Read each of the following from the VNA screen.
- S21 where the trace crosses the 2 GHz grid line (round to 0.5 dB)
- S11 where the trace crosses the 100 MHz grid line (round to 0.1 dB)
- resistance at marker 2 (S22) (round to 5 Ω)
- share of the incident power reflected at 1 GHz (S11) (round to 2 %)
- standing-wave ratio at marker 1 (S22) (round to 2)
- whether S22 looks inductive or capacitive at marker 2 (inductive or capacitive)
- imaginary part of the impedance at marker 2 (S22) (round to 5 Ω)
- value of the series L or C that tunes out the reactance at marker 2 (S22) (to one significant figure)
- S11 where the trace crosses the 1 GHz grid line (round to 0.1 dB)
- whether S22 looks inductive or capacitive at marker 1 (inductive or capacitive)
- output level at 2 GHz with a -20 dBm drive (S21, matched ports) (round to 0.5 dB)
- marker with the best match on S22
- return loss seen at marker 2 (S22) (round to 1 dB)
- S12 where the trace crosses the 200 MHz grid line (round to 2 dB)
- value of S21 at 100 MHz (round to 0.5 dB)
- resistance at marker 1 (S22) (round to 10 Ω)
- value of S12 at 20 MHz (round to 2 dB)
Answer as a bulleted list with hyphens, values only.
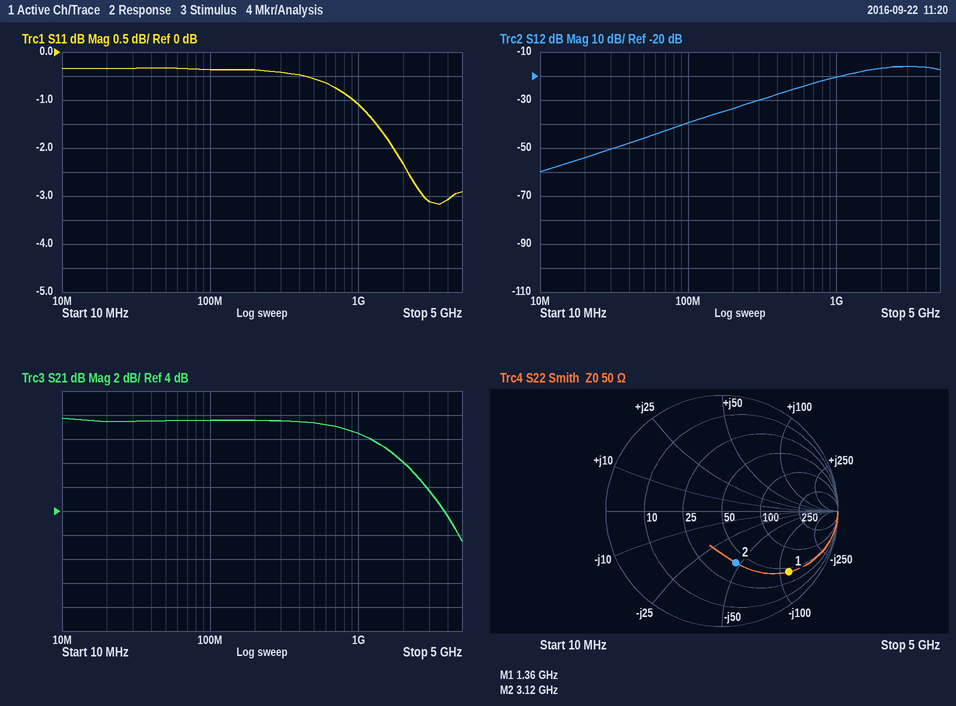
- 8.0 dB
- -0.4 dB
- 40 Ω
- 78 %
- 8
- capacitive
- -45 Ω
- 2 nH
- -1.1 dB
- capacitive
- -12.0 dBm
- marker 2
- 7 dB
- -34 dB
- 11.5 dB
- 40 Ω
- -54 dB
